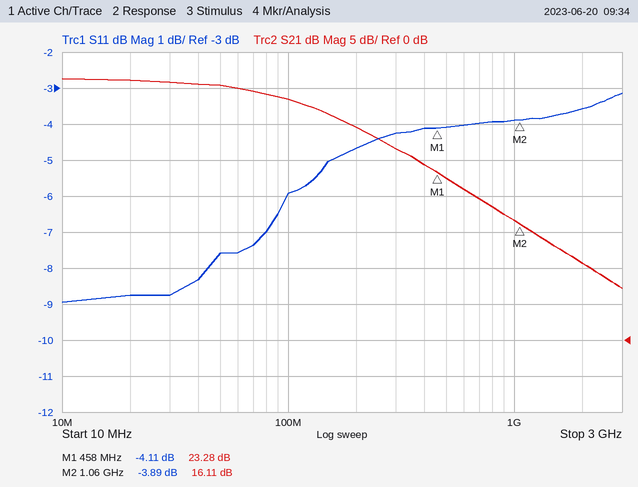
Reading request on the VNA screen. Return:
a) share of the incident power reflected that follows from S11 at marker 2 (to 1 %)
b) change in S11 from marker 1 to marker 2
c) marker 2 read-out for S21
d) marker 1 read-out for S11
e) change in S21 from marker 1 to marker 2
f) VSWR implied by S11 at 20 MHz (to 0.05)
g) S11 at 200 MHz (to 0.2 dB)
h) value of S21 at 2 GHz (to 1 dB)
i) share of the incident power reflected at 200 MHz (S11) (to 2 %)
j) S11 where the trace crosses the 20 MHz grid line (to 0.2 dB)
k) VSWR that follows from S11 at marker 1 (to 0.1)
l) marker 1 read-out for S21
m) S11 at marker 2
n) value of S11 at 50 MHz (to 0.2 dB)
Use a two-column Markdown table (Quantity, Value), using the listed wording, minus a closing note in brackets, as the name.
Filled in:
| Quantity | Value |
|---|---|
| share of the incident power reflected that follows from S11 at marker 2 | 41 % |
| change in S11 from marker 1 to marker 2 | 0.22 dB |
| marker 2 read-out for S21 | 16.11 dB |
| marker 1 read-out for S11 | -4.11 dB |
| change in S21 from marker 1 to marker 2 | -7.17 dB |
| VSWR implied by S11 at 20 MHz | 2.15 |
| S11 at 200 MHz | -4.6 dB |
| value of S21 at 2 GHz | 11 dB |
| share of the incident power reflected at 200 MHz (S11) | 34 % |
| S11 where the trace crosses the 20 MHz grid line | -8.8 dB |
| VSWR that follows from S11 at marker 1 | 4.3 |
| marker 1 read-out for S21 | 23.28 dB |
| S11 at marker 2 | -3.89 dB |
| value of S11 at 50 MHz | -7.6 dB |
